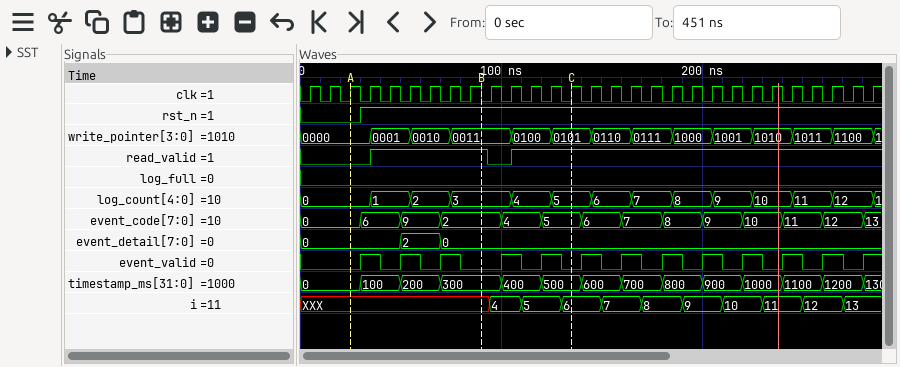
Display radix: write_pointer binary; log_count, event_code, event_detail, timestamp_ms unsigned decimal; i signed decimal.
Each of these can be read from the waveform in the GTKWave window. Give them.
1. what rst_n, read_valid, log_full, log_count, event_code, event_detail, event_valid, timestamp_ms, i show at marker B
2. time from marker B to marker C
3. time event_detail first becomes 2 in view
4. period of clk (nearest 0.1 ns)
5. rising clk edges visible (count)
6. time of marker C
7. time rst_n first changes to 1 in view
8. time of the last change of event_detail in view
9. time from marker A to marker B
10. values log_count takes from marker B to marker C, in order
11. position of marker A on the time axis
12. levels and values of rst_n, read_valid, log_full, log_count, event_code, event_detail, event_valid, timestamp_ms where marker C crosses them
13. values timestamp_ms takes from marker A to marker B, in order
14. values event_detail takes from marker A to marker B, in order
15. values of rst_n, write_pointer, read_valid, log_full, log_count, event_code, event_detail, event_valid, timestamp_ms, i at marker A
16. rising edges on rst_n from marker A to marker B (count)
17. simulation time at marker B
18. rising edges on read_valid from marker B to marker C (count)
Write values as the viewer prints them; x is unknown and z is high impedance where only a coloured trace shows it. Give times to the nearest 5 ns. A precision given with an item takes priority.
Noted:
rst_n=1, read_valid=1, log_full=0, log_count=3, event_code=2, event_detail=0, event_valid=0, timestamp_ms=300, i=XXX
45 ns
50 ns
10 ns
29
135 ns
30 ns
70 ns
65 ns
3, 4, 5
25 ns
rst_n=1, read_valid=1, log_full=0, log_count=5, event_code=5, event_detail=0, event_valid=0, timestamp_ms=500
0, 100, 200, 300
0, 2, 0
rst_n=0, write_pointer=0000, read_valid=0, log_full=0, log_count=0, event_code=0, event_detail=0, event_valid=0, timestamp_ms=0, i=XXX
1
90 ns
1
